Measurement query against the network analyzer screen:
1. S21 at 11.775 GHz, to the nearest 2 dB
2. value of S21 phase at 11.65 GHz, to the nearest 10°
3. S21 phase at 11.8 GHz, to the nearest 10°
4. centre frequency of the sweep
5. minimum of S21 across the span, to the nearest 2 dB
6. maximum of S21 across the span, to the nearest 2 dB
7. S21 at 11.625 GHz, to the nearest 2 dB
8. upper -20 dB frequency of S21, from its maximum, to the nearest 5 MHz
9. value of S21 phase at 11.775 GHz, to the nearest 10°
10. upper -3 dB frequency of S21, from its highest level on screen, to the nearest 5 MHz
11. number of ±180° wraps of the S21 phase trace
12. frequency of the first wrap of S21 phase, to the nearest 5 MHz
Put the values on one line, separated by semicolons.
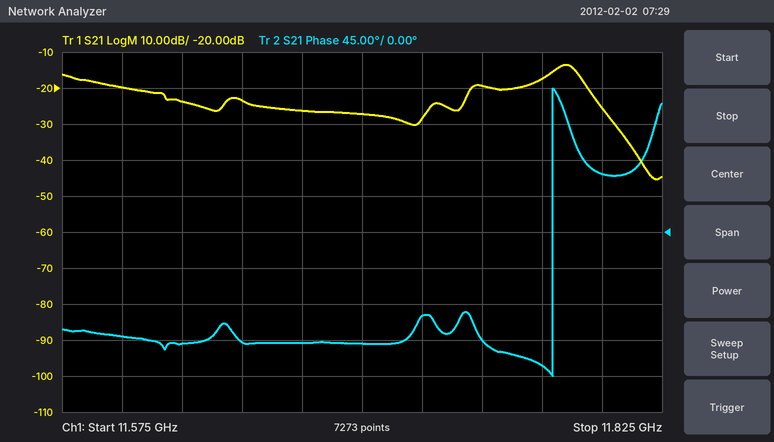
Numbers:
-18 dB; -140°; 70°; 11.7 GHz; -46 dB; -14 dB; -24 dB; 11.810 GHz; -170°; 11.790 GHz; 1; 11.780 GHz
